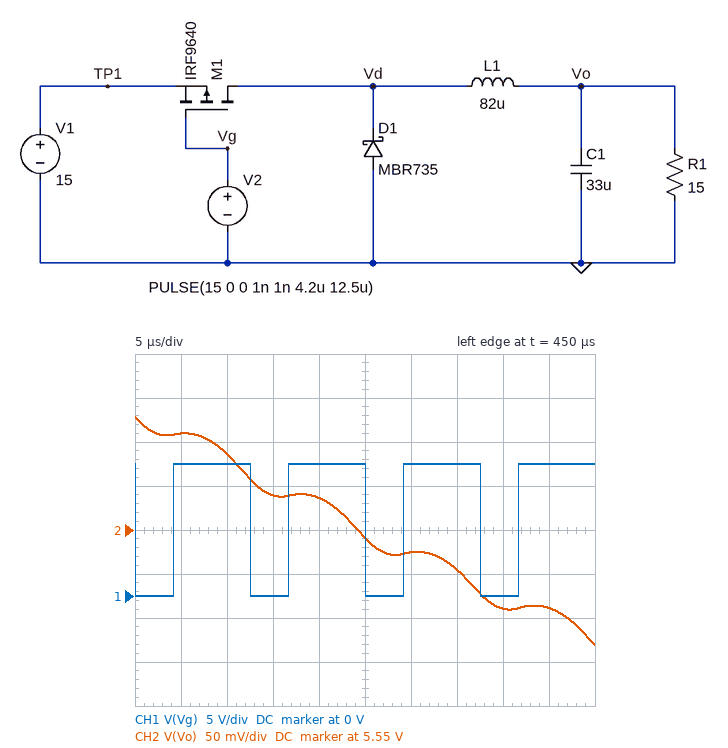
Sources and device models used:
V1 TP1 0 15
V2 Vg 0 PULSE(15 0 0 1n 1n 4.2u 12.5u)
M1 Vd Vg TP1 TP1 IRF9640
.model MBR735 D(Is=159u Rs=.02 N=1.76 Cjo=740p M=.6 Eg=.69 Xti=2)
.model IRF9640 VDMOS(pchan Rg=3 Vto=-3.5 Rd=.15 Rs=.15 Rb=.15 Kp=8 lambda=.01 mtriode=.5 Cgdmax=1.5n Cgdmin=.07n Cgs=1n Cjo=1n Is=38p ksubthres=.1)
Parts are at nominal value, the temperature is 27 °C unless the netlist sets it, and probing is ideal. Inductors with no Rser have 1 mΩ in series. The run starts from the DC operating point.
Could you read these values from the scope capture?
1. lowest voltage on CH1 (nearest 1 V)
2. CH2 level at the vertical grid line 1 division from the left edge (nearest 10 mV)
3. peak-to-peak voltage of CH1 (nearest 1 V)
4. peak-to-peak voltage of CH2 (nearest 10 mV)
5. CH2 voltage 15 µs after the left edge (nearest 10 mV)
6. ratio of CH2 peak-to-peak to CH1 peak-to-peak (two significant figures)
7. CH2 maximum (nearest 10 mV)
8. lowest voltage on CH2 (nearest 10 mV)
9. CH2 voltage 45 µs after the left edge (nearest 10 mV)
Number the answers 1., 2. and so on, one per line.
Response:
1. 0 V
2. 5.66 V
3. 15 V
4. 260 mV
5. 5.59 V
6. 0.017
7. 5.68 V
8. 5.42 V
9. 5.46 V
